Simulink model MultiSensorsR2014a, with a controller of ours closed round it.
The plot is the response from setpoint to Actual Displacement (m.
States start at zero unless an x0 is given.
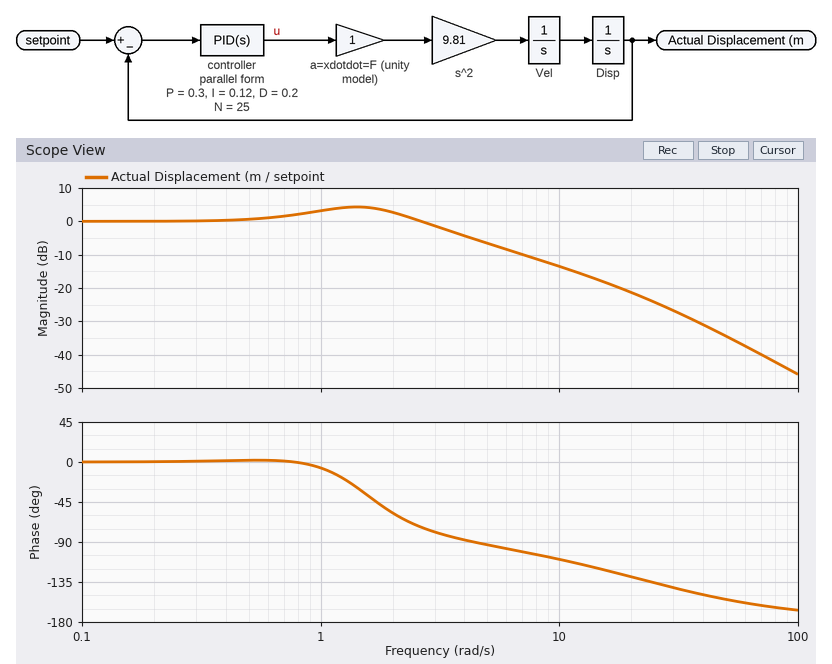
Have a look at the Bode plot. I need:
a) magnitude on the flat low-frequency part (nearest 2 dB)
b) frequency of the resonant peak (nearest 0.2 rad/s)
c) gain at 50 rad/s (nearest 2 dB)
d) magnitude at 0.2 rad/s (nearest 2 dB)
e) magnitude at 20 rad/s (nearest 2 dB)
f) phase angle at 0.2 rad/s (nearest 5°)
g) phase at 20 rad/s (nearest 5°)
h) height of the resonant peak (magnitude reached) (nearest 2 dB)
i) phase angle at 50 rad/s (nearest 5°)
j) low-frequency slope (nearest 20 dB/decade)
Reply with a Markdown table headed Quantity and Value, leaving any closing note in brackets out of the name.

| Quantity | Value |
|---|---|
| magnitude on the flat low-frequency part | 0 dB |
| frequency of the resonant peak | 1.4 rad/s |
| gain at 50 rad/s | -34 dB |
| magnitude at 0.2 rad/s | 0 dB |
| magnitude at 20 rad/s | -22 dB |
| phase angle at 0.2 rad/s | 0° |
| phase at 20 rad/s | -130° |
| height of the resonant peak (magnitude reached) | 4 dB |
| phase angle at 50 rad/s | -155° |
| low-frequency slope | 0 dB/decade |
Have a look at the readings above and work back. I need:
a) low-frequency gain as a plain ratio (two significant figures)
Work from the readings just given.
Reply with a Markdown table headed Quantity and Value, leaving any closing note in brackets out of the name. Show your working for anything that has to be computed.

| Quantity | Value |
|---|---|
| low-frequency gain as a plain ratio | 10^(0 / 20) = 1.0 |
